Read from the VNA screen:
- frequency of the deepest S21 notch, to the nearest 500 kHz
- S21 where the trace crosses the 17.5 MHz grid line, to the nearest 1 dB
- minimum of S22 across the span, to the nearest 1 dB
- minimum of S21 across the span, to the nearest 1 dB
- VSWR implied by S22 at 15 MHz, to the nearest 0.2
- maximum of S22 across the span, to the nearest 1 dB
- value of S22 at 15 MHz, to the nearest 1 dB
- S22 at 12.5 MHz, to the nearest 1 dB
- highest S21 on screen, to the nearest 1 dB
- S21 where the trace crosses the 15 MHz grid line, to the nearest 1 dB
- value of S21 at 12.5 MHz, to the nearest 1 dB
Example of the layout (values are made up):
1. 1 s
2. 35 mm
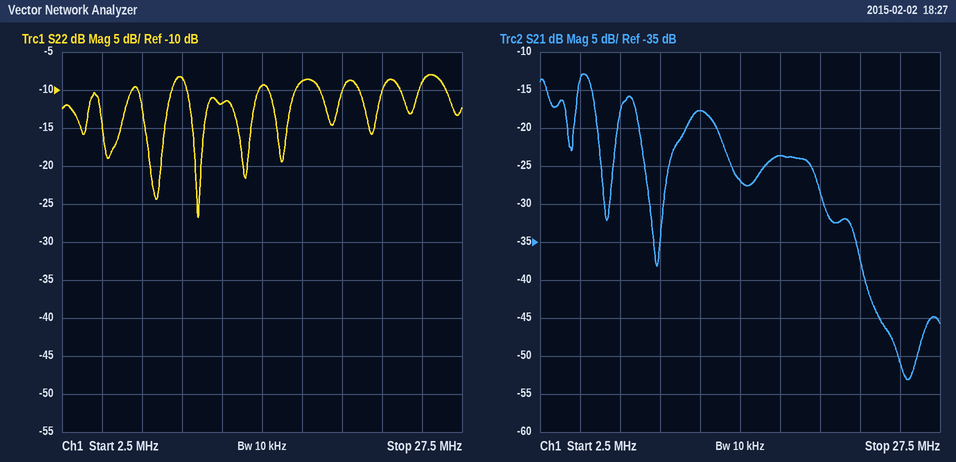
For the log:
1. 25.5 MHz
2. -24 dB
3. -27 dB
4. -53 dB
5. 2.0
6. -8 dB
7. -9 dB
8. -12 dB
9. -13 dB
10. -27 dB
11. -18 dB
